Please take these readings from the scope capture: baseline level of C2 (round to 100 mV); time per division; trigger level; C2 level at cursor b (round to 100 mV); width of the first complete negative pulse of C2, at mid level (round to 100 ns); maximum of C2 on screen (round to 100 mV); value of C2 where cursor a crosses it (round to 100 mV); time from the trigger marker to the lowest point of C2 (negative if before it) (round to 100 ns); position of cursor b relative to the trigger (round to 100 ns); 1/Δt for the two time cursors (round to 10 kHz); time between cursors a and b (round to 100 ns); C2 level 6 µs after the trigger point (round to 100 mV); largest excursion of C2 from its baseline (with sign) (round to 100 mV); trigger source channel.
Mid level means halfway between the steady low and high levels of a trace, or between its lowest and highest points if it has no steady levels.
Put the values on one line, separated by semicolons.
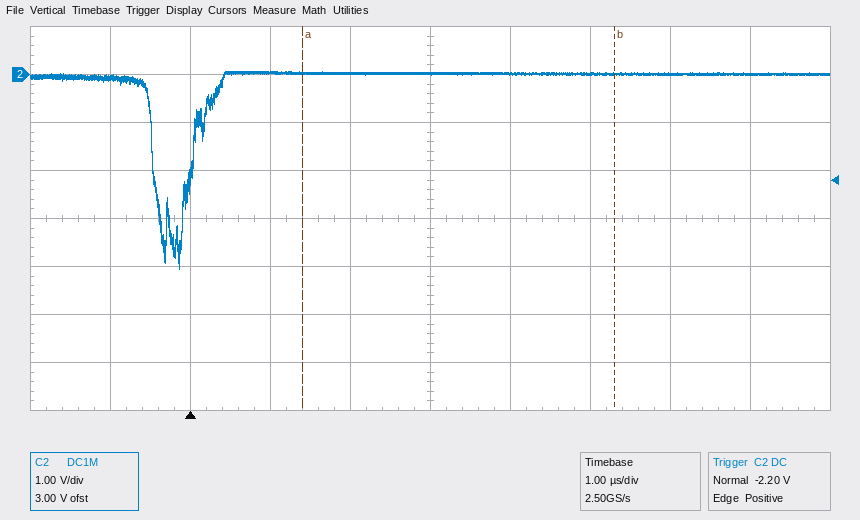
0.0 V; 1 µs; -2.20 V; 0.0 V; 500 ns; 100 mV; 0.0 V; -100 ns; +5.3 µs; 260 kHz; 3.9 µs; 0.0 V; -4.1 V; C2
